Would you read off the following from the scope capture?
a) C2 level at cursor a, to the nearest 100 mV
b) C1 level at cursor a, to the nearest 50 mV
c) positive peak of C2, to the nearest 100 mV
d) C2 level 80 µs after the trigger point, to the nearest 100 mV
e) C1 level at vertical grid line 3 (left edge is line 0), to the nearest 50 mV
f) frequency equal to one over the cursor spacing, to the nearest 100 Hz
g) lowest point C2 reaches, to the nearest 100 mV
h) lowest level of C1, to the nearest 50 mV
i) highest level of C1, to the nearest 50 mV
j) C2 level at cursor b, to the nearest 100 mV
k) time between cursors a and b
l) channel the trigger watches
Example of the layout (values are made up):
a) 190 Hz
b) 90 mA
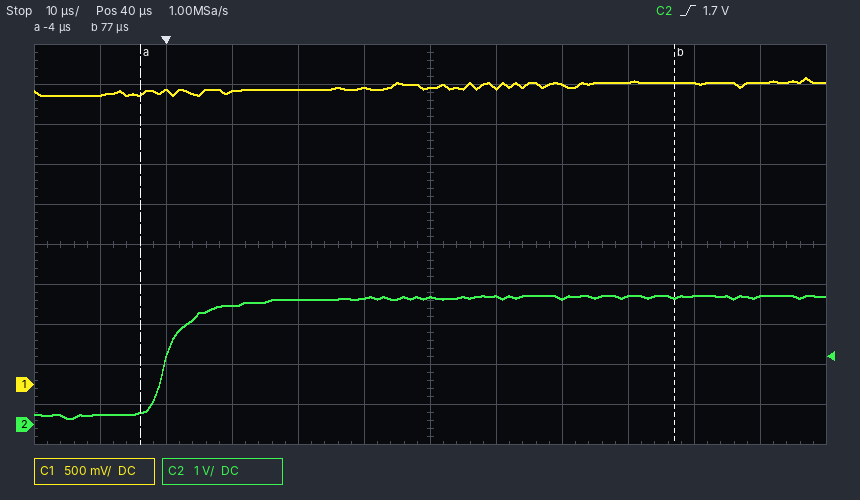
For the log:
a) 300 mV
b) 3.65 V
c) 3.2 V
d) 3.2 V
e) 3.65 V
f) 12.3 kHz
g) 200 mV
h) 3.60 V
i) 3.85 V
j) 3.2 V
k) 81 µs
l) C2
